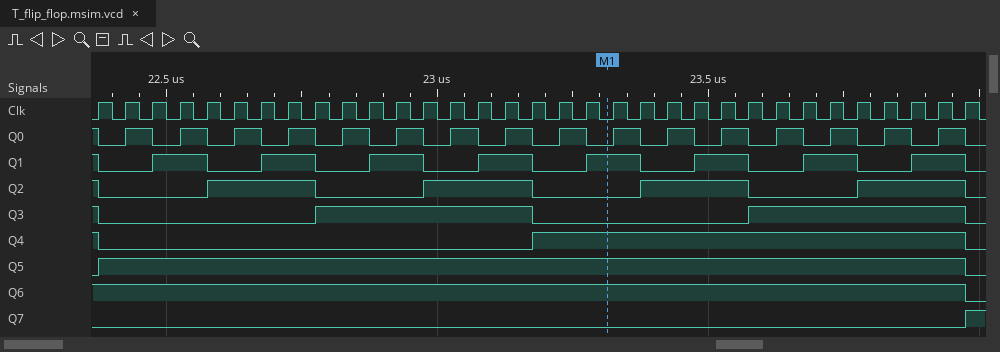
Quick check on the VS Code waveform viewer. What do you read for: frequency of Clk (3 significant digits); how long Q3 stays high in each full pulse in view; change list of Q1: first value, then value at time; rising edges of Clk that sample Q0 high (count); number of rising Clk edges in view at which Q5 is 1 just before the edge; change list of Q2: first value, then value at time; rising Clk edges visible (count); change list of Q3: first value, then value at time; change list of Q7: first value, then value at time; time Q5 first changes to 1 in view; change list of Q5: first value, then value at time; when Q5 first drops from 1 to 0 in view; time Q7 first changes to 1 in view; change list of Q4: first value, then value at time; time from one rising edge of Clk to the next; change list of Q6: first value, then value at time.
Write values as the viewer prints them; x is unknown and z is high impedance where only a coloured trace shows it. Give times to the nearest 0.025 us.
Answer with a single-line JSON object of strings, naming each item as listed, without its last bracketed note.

{"frequency of Clk": "20.0 MHz", "how long Q3 stays high in each full pulse in view": "0.4 us, 0.4 us", "change list of Q1: first value, then value at time": "1, 0 at 22.375 us, 1 at 22.475 us, 0 at 22.575 us, 1 at 22.675 us, 0 at 22.775 us, 1 at 22.875 us, 0 at 22.975 us, 1 at 23.075 us, 0 at 23.175 us, 1 at 23.275 us, 0 at 23.375 us, 1 at 23.475 us, 0 at 23.575 us, 1 at 23.675 us, 0 at 23.775 us, 1 at 23.875 us, 0 at 23.975 us", "rising edges of Clk that sample Q0 high": "17", "number of rising Clk edges in view at which Q5 is 1 just before the edge": "32", "change list of Q2: first value, then value at time": "1, 0 at 22.375 us, 1 at 22.575 us, 0 at 22.775 us, 1 at 22.975 us, 0 at 23.175 us, 1 at 23.375 us, 0 at 23.575 us, 1 at 23.775 us, 0 at 23.975 us", "rising Clk edges visible": "33", "change list of Q3: first value, then value at time": "1, 0 at 22.375 us, 1 at 22.775 us, 0 at 23.175 us, 1 at 23.575 us, 0 at 23.975 us", "change list of Q7: first value, then value at time": "0, 1 at 23.975 us", "time Q5 first changes to 1 in view": "22.375 us", "change list of Q5: first value, then value at time": "0, 1 at 22.375 us, 0 at 23.975 us", "when Q5 first drops from 1 to 0 in view": "23.975 us", "time Q7 first changes to 1 in view": "23.975 us", "change list of Q4: first value, then value at time": "1, 0 at 22.375 us, 1 at 23.175 us, 0 at 23.975 us", "time from one rising edge of Clk to the next": "0.05 us", "change list of Q6: first value, then value at time": "1, 0 at 23.975 us"}
